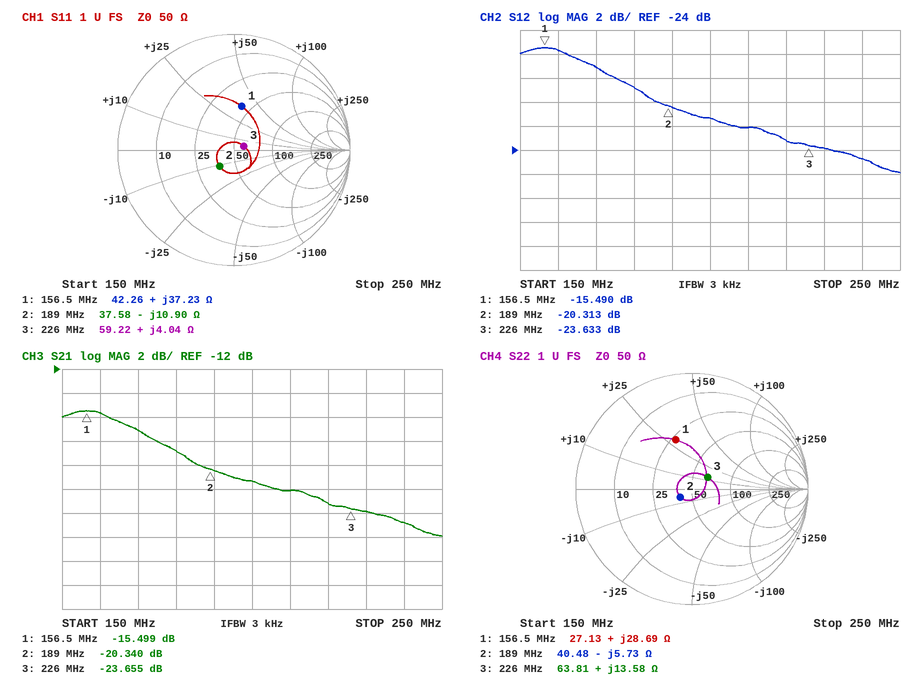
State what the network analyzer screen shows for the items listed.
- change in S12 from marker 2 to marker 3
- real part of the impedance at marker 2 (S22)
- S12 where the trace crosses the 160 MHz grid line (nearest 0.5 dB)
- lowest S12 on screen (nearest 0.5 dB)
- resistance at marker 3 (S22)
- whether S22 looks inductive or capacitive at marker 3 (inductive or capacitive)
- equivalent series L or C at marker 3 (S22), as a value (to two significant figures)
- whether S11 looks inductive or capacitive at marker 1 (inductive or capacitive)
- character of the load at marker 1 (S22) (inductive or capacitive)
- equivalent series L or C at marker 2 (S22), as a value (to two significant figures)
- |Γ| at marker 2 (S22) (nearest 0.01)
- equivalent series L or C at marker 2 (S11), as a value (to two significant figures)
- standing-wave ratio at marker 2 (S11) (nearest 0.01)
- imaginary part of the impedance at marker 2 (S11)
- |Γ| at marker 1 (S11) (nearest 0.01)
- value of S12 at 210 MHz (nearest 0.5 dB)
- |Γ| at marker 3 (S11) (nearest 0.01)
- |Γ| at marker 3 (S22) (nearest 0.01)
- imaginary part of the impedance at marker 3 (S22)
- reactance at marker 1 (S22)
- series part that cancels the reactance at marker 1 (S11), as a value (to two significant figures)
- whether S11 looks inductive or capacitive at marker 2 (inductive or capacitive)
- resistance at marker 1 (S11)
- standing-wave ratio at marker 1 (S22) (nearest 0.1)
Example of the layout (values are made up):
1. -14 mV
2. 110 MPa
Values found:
1. -3.320 dB
2. 40.48 Ω
3. -15.5 dB
4. -26.0 dB
5. 63.81 Ω
6. inductive
7. 9.6 nH
8. inductive
9. inductive
10. 150 pF
11. 0.12
12. 77 pF
13. 1.46
14. -10.90 Ω
15. 0.38
16. -22.0 dB
17. 0.09
18. 0.17
19. +13.58 Ω
20. +28.69 Ω
21. 27 pF
22. capacitive
23. 42.26 Ω
24. 2.6
